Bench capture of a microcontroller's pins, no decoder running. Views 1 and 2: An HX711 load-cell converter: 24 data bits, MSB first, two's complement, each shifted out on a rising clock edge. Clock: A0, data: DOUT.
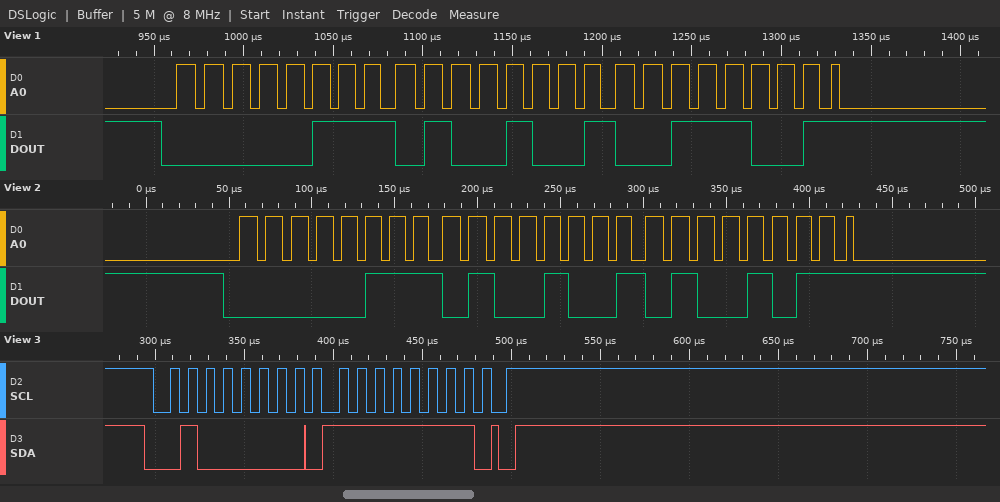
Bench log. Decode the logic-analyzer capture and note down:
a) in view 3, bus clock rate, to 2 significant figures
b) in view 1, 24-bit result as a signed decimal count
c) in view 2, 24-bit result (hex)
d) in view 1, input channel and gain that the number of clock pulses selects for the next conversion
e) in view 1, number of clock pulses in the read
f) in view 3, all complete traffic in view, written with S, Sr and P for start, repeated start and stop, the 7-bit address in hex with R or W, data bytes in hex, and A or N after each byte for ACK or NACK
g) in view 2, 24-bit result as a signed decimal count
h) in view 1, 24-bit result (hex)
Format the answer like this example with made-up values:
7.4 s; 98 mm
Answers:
100 kHz; 477497; 0x07494B; channel A, gain 128; 25; S 20W A FF A P; 477515; 0x074939
